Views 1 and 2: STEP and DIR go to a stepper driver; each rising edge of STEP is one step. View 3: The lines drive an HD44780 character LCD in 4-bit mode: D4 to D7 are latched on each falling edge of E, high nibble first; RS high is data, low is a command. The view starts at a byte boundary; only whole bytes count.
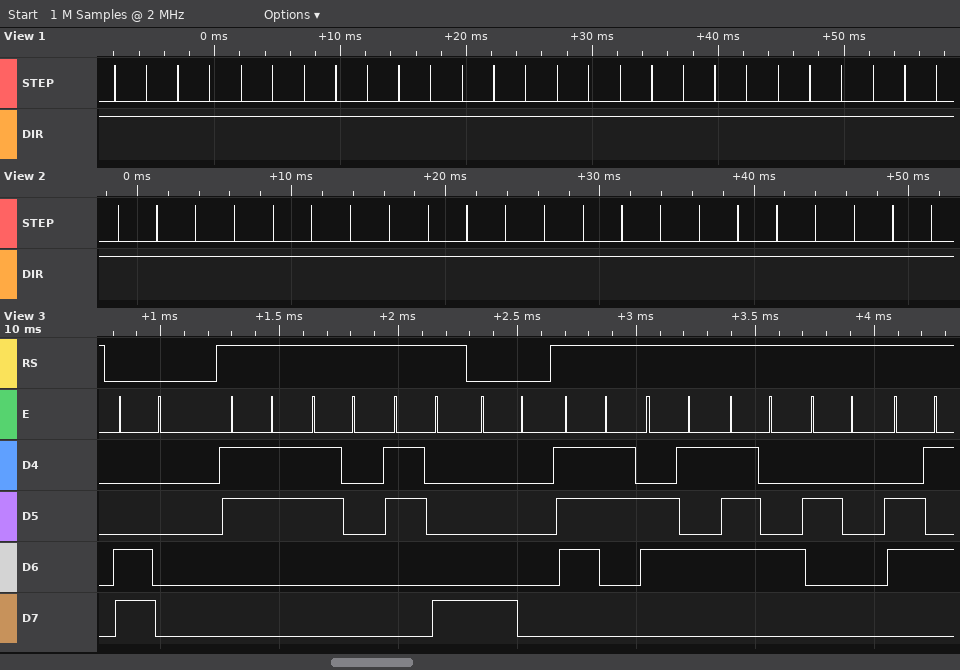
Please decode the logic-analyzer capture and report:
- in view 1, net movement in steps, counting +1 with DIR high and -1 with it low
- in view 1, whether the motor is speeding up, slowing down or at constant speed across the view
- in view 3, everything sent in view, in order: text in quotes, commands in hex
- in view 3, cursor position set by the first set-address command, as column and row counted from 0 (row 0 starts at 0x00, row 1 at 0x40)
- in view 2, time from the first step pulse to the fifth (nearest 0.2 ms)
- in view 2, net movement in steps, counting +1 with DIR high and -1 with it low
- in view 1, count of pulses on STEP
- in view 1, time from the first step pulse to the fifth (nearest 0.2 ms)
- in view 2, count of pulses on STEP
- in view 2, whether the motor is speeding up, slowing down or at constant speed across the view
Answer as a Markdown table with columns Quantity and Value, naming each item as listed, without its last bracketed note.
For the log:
| Quantity | Value |
|---|---|
| in view 1, net movement in steps, counting +1 with DIR high and -1 with it low | +27 |
| in view 1, whether the motor is speeding up, slowing down or at constant speed across the view | constant speed |
| in view 3, everything sent in view, in order: text in quotes, commands in hex | 0xC0 "308" 0x80 "set e" |
| in view 3, cursor position set by the first set-address command, as column and row counted from 0 | column 0, row 1 |
| in view 2, time from the first step pulse to the fifth | 10.0 ms |
| in view 2, net movement in steps, counting +1 with DIR high and -1 with it low | +22 |
| in view 1, count of pulses on STEP | 27 |
| in view 1, time from the first step pulse to the fifth | 10.0 ms |
| in view 2, count of pulses on STEP | 22 |
| in view 2, whether the motor is speeding up, slowing down or at constant speed across the view | constant speed |
